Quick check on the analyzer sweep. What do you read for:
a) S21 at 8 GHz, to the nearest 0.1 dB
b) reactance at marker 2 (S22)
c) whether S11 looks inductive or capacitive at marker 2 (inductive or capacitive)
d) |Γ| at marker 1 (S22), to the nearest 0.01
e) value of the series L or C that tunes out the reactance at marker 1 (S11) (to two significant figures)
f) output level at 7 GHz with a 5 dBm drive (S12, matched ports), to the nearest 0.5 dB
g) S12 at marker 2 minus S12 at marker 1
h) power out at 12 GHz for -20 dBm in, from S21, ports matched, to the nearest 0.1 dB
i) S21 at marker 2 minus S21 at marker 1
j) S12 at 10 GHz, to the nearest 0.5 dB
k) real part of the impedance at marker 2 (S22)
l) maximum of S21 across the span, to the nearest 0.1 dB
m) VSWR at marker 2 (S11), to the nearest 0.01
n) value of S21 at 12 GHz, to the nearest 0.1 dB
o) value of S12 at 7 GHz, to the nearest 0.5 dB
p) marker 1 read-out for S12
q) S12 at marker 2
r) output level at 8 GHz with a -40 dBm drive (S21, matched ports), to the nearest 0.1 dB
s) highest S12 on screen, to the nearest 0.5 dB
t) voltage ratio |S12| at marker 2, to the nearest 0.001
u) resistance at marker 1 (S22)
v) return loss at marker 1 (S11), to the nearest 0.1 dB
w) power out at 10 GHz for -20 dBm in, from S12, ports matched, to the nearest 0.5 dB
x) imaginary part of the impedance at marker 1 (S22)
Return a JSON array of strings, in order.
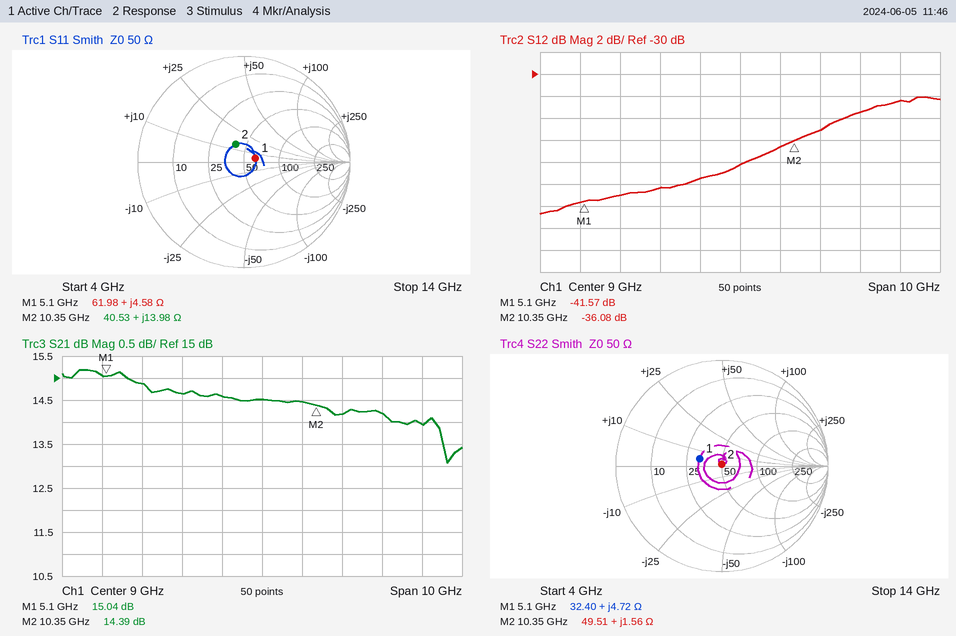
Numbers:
["14.6 dB", "+1.56 Ω", "inductive", "0.22", "6.8 pF", "-35.5 dBm", "5.49 dB", "-5.8 dBm", "-0.65 dB", "-36.5 dB", "49.51 Ω", "15.2 dB", "1.45", "14.2 dB", "-40.5 dB", "-41.57 dB", "-36.08 dB", "-25.4 dBm", "-32.0 dB", "0.016", "32.40 Ω", "18.8 dB", "-56.5 dBm", "+4.72 Ω"]
